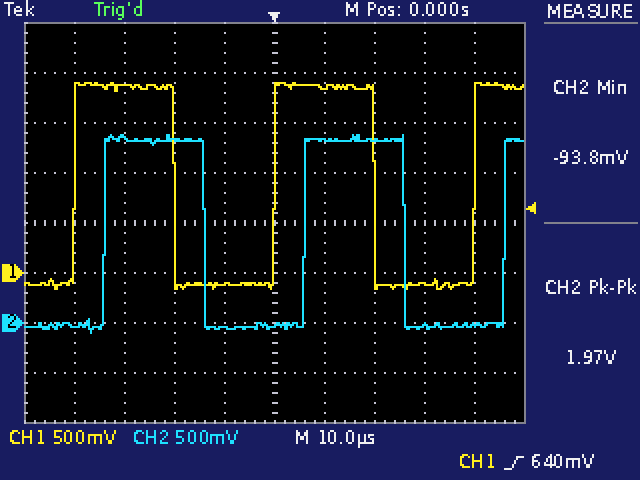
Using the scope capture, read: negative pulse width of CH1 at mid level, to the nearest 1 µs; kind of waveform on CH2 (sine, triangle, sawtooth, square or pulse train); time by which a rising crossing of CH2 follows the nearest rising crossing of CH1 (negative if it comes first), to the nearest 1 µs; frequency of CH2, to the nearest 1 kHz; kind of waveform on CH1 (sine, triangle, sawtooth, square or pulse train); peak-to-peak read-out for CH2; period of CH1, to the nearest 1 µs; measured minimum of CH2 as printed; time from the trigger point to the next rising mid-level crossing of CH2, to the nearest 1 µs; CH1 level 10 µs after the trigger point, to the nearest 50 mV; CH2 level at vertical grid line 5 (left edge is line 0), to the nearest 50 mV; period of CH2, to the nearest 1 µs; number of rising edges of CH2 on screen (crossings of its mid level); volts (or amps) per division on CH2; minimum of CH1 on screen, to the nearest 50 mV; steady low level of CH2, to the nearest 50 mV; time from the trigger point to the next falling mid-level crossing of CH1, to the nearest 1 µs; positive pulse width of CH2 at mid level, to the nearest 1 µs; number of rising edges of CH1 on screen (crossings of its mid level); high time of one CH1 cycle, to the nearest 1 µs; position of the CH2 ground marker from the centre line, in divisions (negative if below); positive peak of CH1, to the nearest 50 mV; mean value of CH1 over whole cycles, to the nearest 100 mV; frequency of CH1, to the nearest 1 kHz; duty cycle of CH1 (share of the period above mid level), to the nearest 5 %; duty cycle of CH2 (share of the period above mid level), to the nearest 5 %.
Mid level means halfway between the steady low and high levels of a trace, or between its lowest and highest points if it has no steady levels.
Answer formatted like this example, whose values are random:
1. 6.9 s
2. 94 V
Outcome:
1. 20 µs
2. square
3. +6 µs
4. 25 kHz
5. square
6. 1.97 V
7. 40 µs
8. -93.8 mV
9. 6 µs
10. 1.85 V
11. 0 mV
12. 40 µs
13. 3
14. 500 mV
15. -150 mV
16. -50 mV
17. 20 µs
18. 20 µs
19. 3
20. 20 µs
21. -2.0 div
22. 1.90 V
23. 900 mV
24. 25 kHz
25. 50 %
26. 50 %
